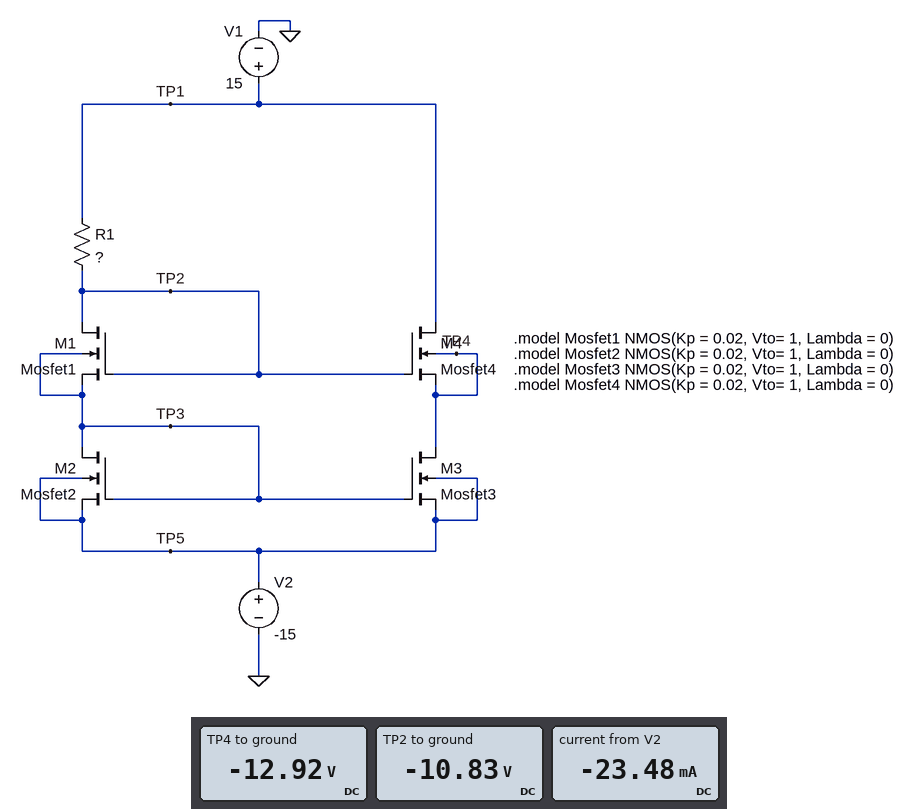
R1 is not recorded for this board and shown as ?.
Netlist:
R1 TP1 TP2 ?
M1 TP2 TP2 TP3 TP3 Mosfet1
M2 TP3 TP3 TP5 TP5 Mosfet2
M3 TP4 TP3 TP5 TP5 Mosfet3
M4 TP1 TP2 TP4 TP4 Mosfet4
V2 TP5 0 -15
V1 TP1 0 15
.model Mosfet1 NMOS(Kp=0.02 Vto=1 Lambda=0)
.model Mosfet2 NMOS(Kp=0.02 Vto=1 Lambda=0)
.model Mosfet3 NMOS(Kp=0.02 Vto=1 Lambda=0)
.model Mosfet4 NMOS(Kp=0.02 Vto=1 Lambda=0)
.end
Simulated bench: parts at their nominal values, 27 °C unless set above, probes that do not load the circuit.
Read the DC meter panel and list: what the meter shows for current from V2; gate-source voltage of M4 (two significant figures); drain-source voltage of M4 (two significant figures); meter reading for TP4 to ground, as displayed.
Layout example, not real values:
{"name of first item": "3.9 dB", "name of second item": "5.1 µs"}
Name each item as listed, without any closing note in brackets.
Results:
{"what the meter shows for current from V2": "-23.48 mA", "gate-source voltage of M4": "2.1 V", "drain-source voltage of M4": "28 V", "meter reading for TP4 to ground, as displayed": "-12.92 V"}
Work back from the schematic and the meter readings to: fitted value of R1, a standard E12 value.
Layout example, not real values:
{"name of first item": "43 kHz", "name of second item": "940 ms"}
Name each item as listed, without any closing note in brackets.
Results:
{"fitted value of R1, a standard E12 value": "2.2 kΩ"}
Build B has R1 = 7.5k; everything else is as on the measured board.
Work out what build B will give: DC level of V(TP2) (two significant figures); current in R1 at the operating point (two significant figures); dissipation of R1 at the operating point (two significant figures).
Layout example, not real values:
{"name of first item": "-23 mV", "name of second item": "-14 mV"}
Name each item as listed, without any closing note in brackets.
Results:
{"DC level of V(TP2)": "-12 V", "current in R1 at the operating point": "3.6 mA", "dissipation of R1 at the operating point": "96 mW"}
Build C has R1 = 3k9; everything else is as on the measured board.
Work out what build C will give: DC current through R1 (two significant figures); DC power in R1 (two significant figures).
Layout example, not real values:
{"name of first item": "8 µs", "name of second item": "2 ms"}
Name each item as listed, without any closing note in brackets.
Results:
{"DC current through R1": "6.8 mA", "DC power in R1": "180 mW"}
